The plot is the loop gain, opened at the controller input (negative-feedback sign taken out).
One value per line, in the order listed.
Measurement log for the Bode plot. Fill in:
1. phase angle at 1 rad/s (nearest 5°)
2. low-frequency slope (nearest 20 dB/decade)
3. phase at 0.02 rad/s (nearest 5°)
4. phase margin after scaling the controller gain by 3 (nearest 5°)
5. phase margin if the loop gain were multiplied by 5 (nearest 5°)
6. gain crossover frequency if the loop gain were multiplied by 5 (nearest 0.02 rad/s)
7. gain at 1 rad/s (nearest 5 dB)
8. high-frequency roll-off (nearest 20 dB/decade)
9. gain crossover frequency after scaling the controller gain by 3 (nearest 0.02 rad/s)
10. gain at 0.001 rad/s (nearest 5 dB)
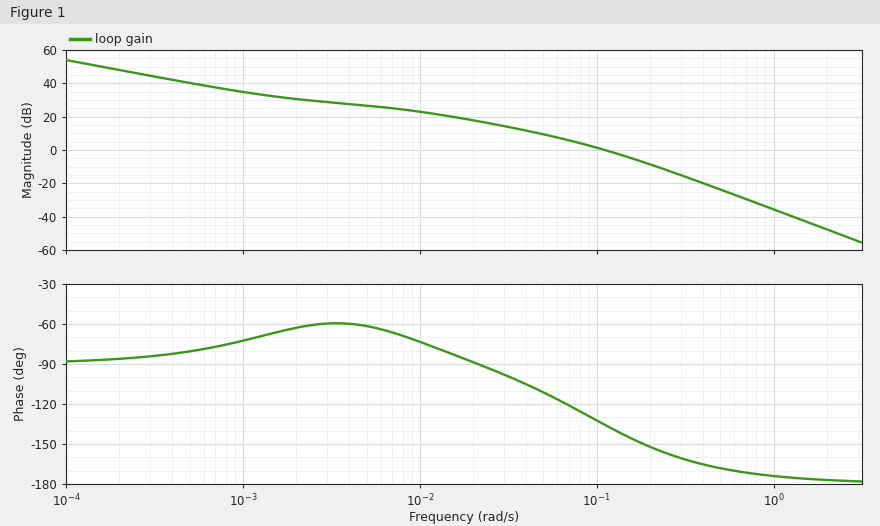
-175°
-20 dB/decade
-90°
25°
20°
0.28 rad/s
-35 dB
-40 dB/decade
0.22 rad/s
35 dB
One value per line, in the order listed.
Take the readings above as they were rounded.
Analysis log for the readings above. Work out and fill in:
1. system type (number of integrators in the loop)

1
